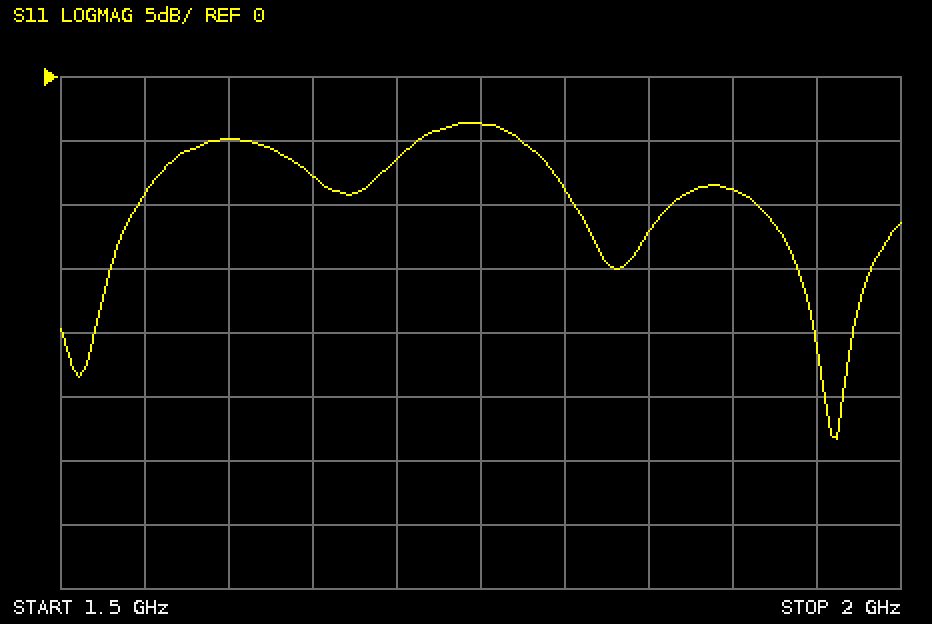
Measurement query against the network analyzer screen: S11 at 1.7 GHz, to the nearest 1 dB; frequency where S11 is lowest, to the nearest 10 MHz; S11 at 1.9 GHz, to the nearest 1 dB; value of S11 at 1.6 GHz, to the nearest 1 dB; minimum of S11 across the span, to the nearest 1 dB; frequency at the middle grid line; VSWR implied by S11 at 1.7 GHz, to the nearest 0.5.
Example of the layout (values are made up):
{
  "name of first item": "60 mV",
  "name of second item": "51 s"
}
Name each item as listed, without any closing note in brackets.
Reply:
{
  "S11 at 1.7 GHz, to the nearest 1 dB": "-6 dB",
  "frequency where S11 is lowest, to the nearest 10 MHz": "1.96 GHz",
  "S11 at 1.9 GHz, to the nearest 1 dB": "-9 dB",
  "value of S11 at 1.6 GHz, to the nearest 1 dB": "-5 dB",
  "minimum of S11 across the span, to the nearest 1 dB": "-28 dB",
  "frequency at the middle grid line": "1.75 GHz",
  "VSWR implied by S11 at 1.7 GHz, to the nearest 0.5": "3.0"
}
